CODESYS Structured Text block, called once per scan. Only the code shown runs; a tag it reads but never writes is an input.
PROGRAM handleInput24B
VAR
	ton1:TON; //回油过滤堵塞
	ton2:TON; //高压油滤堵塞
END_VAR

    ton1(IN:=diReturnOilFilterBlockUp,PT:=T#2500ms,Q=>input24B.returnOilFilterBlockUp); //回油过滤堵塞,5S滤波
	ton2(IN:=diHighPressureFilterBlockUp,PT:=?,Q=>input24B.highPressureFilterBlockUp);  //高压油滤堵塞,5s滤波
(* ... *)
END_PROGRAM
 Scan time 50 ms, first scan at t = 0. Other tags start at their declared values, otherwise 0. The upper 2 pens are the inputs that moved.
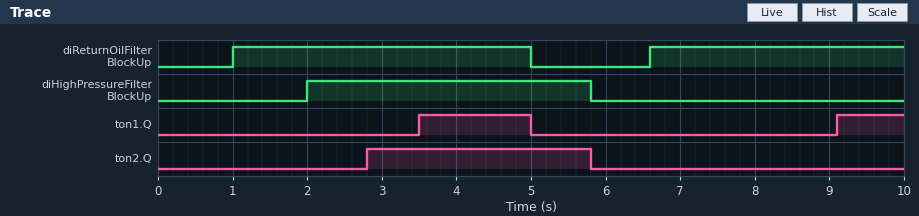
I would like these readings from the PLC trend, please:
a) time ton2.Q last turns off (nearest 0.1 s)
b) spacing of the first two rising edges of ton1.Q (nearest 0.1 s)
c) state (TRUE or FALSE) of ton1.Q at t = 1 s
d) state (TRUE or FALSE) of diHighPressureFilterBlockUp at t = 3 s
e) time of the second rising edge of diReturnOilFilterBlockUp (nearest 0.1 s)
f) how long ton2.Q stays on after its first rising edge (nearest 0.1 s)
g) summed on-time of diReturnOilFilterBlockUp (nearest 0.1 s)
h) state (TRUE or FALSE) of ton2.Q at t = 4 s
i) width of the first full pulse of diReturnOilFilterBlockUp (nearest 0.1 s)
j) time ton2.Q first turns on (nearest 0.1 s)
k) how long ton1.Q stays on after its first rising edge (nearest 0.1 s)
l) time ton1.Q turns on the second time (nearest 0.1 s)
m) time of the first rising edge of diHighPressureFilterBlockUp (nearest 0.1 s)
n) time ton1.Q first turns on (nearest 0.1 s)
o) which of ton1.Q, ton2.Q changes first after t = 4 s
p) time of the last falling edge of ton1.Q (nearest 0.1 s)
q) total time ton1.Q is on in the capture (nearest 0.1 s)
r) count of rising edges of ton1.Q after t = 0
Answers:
5.8 s
5.6 s
FALSE
TRUE
6.6 s
3.0 s
7.4 s
TRUE
4.0 s
2.8 s
1.5 s
9.1 s
2.0 s
3.5 s
ton1.Q
5.0 s
2.4 s
2
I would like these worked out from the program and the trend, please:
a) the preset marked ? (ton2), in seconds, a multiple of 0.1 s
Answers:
0.8 s
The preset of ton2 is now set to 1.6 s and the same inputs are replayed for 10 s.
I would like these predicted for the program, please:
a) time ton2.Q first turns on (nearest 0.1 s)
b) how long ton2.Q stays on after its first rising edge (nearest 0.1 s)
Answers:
3.6 s
2.2 s
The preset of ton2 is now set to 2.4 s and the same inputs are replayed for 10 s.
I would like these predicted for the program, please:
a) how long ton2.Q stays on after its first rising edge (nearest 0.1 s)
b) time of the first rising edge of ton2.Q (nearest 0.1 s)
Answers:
1.4 s
4.4 s
